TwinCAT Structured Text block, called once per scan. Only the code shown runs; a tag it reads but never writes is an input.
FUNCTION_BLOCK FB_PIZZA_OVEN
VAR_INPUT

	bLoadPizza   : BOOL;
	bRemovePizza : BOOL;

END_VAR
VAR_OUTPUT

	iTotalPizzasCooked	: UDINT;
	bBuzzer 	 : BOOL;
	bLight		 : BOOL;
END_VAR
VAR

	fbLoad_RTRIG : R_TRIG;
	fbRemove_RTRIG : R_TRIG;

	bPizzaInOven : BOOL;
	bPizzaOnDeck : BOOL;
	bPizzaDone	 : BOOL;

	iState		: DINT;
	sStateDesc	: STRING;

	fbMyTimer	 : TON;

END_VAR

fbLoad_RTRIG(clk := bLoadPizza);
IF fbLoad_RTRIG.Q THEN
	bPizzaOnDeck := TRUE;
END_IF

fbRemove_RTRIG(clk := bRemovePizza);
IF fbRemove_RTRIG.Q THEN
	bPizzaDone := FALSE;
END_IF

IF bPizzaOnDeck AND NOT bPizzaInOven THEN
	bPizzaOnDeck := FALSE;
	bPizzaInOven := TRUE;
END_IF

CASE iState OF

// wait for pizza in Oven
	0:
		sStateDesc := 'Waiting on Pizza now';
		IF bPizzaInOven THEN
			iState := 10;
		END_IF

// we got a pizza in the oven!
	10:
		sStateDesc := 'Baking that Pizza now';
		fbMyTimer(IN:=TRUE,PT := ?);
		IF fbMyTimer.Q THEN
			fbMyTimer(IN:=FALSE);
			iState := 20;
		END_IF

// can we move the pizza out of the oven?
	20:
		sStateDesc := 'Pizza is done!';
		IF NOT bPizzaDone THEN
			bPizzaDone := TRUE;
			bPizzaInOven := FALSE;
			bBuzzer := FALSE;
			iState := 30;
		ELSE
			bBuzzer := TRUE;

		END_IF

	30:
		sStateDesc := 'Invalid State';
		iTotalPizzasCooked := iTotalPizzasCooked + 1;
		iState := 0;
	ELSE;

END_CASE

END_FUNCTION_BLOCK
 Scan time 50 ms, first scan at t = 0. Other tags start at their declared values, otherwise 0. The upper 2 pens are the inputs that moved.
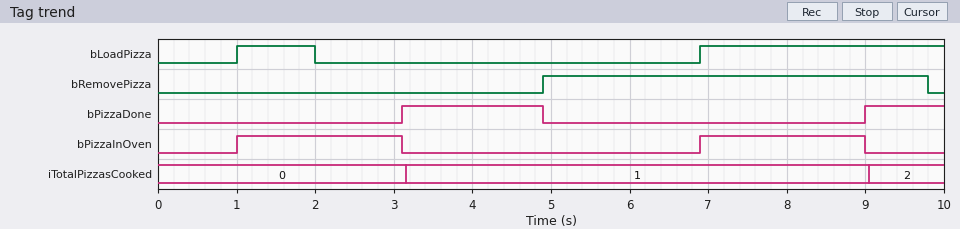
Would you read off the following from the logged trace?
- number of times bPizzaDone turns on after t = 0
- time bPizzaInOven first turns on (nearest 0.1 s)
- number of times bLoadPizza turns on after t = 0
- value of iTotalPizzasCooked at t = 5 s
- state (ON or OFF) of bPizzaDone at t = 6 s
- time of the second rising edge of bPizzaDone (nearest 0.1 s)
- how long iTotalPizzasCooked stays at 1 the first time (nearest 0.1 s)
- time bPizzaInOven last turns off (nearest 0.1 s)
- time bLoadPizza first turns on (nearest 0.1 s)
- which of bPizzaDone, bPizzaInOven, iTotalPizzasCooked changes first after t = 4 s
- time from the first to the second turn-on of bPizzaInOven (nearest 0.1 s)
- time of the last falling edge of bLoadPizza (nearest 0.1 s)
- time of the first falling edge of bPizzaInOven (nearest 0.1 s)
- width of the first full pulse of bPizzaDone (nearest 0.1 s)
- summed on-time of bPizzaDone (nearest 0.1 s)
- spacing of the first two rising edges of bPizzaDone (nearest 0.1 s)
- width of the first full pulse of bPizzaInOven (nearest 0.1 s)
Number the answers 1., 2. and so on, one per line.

1. 2
2. 1.0 s
3. 2
4. 1
5. OFF
6. 9.0 s
7. 5.9 s
8. 9.0 s
9. 1.0 s
10. bPizzaDone
11. 5.9 s
12. 2.0 s
13. 3.1 s
14. 1.8 s
15. 2.8 s
16. 5.9 s
17. 2.1 s
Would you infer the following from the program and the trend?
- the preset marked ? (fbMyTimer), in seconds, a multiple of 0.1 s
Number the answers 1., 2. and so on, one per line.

1. 2.0 s
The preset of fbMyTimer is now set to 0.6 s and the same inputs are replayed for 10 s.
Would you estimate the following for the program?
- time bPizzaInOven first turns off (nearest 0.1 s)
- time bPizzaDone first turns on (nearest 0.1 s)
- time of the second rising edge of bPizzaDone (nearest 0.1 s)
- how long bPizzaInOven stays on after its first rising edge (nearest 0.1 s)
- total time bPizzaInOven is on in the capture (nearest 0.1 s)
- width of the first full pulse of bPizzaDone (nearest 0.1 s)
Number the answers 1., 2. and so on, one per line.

1. 1.7 s
2. 1.7 s
3. 7.6 s
4. 0.7 s
5. 1.4 s
6. 3.2 s
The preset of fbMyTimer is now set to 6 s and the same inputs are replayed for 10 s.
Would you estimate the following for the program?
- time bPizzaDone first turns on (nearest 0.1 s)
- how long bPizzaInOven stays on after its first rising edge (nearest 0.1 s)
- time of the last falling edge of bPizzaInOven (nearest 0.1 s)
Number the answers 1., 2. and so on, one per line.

1. 7.1 s
2. 6.1 s
3. 7.1 s
